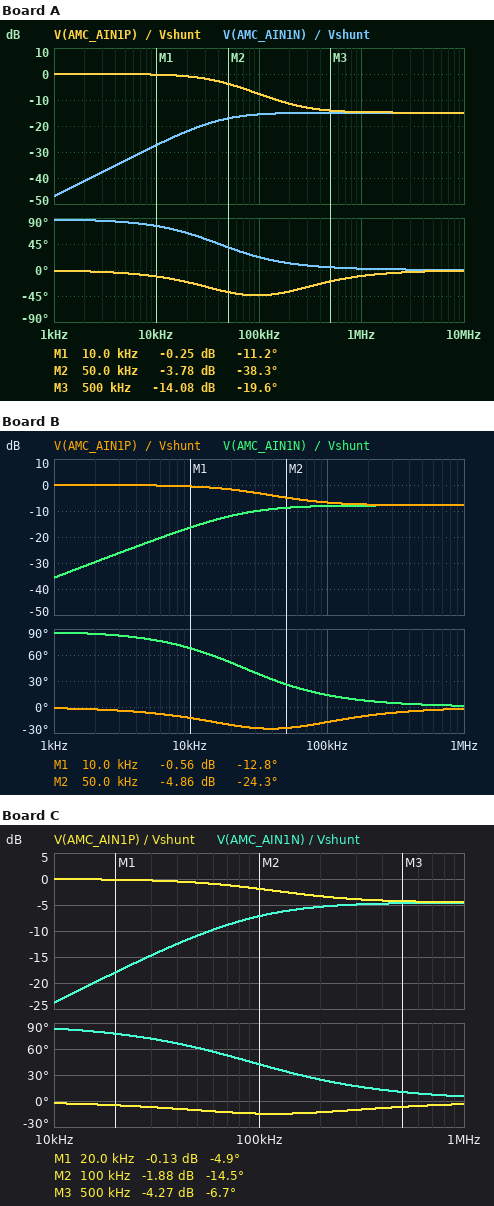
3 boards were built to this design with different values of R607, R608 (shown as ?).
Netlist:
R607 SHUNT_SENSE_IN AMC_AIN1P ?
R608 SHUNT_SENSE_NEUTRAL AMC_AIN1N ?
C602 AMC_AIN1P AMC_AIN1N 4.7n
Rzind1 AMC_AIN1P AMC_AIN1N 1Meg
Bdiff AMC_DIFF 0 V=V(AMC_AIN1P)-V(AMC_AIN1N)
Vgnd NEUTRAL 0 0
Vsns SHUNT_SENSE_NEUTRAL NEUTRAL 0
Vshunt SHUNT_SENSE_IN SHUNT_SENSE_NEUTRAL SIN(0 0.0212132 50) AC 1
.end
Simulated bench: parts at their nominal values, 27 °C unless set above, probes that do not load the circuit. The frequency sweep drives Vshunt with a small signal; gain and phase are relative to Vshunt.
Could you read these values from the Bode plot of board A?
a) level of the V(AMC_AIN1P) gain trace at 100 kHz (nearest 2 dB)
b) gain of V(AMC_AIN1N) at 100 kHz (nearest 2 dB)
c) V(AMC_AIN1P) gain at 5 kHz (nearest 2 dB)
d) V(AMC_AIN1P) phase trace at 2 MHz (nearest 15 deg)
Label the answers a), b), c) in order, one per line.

a) -8 dB
b) -16 dB
c) 0 dB
d) 0 deg
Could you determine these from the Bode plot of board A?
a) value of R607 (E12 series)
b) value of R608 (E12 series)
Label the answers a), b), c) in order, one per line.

a) 680 Ω
b) 150 Ω
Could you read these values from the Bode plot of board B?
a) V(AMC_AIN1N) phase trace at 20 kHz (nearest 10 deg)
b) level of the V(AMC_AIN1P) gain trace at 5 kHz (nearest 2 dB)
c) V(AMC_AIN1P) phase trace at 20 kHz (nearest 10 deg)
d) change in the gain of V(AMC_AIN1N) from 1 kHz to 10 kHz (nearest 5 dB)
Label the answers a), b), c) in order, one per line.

a) 50 deg
b) 0 dB
c) -20 deg
d) 20 dB
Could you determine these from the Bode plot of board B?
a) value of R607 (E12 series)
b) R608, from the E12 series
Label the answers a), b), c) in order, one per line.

a) 820 Ω
b) 560 Ω
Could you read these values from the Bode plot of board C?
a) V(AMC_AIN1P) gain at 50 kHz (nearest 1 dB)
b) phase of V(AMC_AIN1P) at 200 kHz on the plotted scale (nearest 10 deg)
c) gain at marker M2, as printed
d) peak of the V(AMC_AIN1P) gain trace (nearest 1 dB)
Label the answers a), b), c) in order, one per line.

a) -1 dB
b) -10 deg
c) -1.88 dB
d) 0 dB
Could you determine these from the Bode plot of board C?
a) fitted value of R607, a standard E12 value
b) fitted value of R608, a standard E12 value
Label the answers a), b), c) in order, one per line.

a) 150 Ω
b) 220 Ω
